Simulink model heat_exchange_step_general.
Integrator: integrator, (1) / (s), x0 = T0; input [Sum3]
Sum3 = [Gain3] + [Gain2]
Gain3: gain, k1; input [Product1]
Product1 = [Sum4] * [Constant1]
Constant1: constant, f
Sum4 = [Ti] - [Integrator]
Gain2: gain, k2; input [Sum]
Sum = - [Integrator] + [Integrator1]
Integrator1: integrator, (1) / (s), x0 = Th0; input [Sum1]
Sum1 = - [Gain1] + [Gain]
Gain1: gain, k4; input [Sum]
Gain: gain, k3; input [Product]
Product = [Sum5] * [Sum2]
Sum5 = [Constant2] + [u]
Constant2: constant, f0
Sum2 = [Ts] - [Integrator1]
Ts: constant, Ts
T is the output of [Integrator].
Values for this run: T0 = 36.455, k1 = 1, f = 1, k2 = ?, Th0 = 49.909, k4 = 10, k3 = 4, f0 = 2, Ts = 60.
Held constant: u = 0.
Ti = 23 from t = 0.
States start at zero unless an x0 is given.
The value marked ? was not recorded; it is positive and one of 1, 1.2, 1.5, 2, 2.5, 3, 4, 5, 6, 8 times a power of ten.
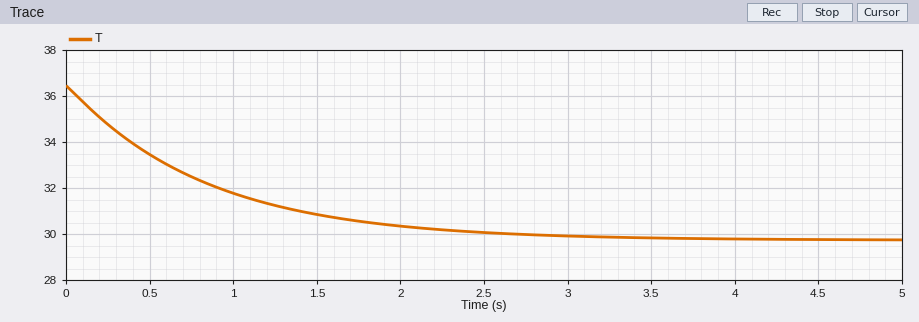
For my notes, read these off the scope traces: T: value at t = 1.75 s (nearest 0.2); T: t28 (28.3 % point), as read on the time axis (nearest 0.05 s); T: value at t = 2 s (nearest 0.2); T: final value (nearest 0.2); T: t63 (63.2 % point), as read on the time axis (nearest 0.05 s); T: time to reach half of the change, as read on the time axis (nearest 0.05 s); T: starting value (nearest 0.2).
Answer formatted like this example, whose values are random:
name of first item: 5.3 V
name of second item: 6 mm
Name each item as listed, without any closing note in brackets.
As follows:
T: value at t = 1.75 s: 30.6
T: t28 (28.3 % point), as read on the time axis: 0.30 s
T: value at t = 2 s: 30.4
T: final value: 29.8
T: t63 (63.2 % point), as read on the time axis: 0.85 s
T: time to reach half of the change, as read on the time axis: 0.60 s
T: starting value: 36.4
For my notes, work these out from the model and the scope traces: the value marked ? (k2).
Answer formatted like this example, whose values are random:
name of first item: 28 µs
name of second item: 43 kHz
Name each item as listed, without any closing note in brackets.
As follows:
the value marked ?: 0.5
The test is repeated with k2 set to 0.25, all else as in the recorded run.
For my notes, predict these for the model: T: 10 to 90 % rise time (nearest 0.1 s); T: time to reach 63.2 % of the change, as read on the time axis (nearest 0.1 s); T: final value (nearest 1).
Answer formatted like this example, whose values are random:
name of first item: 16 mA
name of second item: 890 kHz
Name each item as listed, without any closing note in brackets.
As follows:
T: 10 to 90 % rise time: 2.0 s
T: time to reach 63.2 % of the change, as read on the time axis: 0.9 s
T: final value: 27
